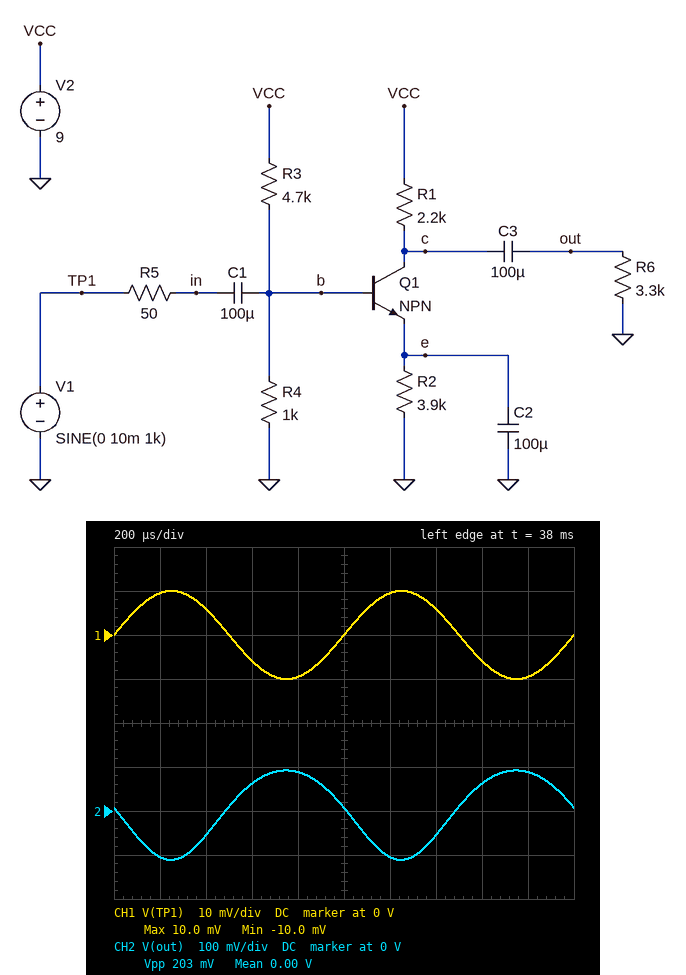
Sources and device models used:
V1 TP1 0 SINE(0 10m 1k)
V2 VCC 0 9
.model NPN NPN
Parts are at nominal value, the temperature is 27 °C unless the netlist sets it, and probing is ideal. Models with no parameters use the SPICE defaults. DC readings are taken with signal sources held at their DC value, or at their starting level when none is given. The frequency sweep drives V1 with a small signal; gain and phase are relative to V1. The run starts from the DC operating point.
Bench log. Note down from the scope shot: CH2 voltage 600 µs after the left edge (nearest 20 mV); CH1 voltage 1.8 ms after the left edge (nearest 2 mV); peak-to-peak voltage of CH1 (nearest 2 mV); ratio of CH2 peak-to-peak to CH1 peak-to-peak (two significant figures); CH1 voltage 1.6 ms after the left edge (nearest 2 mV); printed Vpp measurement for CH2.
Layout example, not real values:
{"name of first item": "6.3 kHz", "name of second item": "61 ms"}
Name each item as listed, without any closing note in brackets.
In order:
{"CH2 voltage 600 µs after the left edge": "60 mV", "CH1 voltage 1.8 ms after the left edge": "-10 mV", "peak-to-peak voltage of CH1": "20 mV", "ratio of CH2 peak-to-peak to CH1 peak-to-peak": "10", "CH1 voltage 1.6 ms after the left edge": "-6 mV", "printed Vpp measurement for CH2": "203 mV"}
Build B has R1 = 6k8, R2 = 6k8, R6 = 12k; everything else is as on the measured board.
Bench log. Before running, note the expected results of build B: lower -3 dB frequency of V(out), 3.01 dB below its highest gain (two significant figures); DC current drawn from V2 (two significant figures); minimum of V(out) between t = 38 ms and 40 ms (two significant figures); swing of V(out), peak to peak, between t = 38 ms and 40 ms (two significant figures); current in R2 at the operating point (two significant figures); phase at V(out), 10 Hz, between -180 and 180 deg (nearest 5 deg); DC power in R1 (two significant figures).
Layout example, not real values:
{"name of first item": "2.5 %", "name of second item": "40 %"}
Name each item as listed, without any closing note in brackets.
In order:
{"lower -3 dB frequency of V(out), 3.01 dB below its highest gain": "8.4 Hz", "DC current drawn from V2": "1.7 mA", "minimum of V(out) between t = 38 ms and 40 ms": "-220 mV", "swing of V(out), peak to peak, between t = 38 ms and 40 ms": "390 mV", "current in R2 at the operating point": "130 µA", "phase at V(out), 10 Hz, between -180 and 180 deg": "-130 deg", "DC power in R1": "110 µW"}
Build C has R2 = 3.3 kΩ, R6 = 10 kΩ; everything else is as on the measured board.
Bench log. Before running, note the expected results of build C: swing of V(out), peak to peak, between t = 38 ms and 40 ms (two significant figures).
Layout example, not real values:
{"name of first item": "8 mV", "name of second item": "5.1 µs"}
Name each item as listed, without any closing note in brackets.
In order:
{"swing of V(out), peak to peak, between t = 38 ms and 40 ms": "330 mV"}
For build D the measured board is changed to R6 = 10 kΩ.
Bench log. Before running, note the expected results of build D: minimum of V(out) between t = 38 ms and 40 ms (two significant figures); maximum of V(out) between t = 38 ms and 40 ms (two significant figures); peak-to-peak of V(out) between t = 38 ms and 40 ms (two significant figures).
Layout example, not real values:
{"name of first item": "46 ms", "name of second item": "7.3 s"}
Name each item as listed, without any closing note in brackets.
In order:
{"minimum of V(out) between t = 38 ms and 40 ms": "-150 mV", "maximum of V(out) between t = 38 ms and 40 ms": "130 mV", "peak-to-peak of V(out) between t = 38 ms and 40 ms": "280 mV"}
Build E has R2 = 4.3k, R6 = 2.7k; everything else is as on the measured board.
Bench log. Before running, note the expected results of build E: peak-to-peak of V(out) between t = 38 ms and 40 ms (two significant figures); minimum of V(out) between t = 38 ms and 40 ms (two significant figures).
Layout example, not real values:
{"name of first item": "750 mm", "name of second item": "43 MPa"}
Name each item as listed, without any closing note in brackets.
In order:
{"peak-to-peak of V(out) between t = 38 ms and 40 ms": "170 mV", "minimum of V(out) between t = 38 ms and 40 ms": "-93 mV"}
